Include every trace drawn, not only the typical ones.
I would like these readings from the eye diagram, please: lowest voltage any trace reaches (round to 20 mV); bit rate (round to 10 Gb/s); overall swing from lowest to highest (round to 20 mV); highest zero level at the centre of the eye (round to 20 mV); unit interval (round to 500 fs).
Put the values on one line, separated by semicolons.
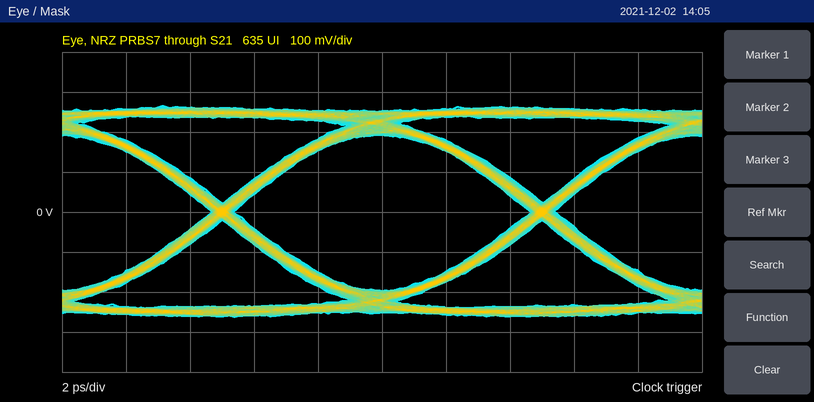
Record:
-260 mV; 100 Gb/s; 520 mV; -200 mV; 10.0 ps
